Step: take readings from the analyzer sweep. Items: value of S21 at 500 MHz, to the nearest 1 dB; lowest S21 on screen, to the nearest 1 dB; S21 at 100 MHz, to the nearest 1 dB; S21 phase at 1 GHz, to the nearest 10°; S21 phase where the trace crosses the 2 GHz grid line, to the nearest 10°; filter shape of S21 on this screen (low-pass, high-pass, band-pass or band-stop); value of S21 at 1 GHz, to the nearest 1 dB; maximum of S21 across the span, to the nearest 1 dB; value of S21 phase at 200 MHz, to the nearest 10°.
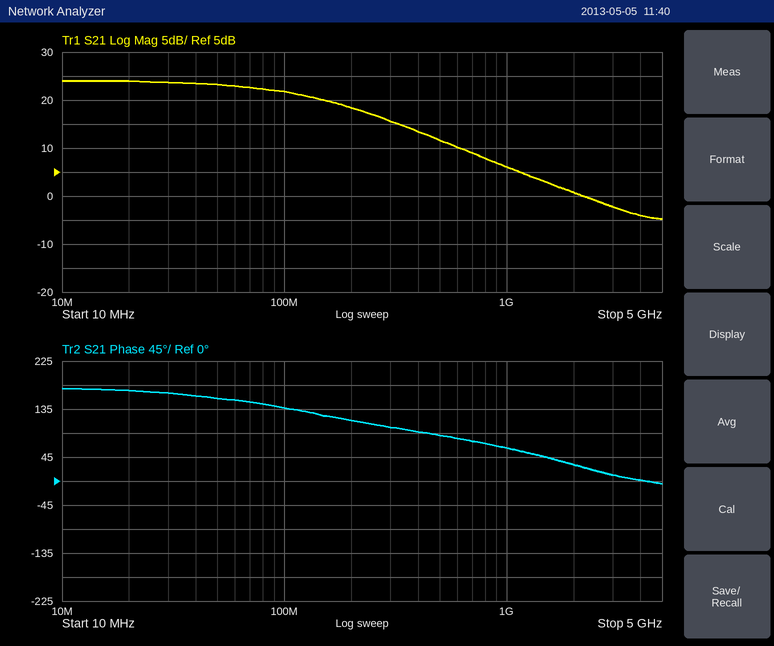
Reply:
12 dB
-5 dB
22 dB
60°
30°
low-pass
6 dB
24 dB
110°
